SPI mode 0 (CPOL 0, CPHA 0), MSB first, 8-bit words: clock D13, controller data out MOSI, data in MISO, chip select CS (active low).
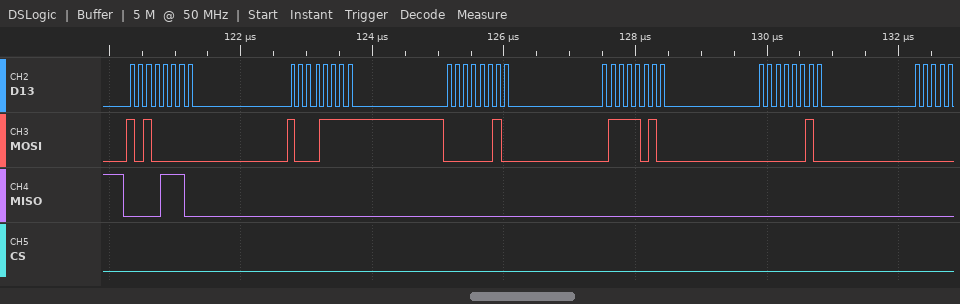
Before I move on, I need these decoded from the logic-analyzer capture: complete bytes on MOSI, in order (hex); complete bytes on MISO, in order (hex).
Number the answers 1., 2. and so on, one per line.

1. A0 8F 02 7A 02
2. 0E 00 00 00 00
